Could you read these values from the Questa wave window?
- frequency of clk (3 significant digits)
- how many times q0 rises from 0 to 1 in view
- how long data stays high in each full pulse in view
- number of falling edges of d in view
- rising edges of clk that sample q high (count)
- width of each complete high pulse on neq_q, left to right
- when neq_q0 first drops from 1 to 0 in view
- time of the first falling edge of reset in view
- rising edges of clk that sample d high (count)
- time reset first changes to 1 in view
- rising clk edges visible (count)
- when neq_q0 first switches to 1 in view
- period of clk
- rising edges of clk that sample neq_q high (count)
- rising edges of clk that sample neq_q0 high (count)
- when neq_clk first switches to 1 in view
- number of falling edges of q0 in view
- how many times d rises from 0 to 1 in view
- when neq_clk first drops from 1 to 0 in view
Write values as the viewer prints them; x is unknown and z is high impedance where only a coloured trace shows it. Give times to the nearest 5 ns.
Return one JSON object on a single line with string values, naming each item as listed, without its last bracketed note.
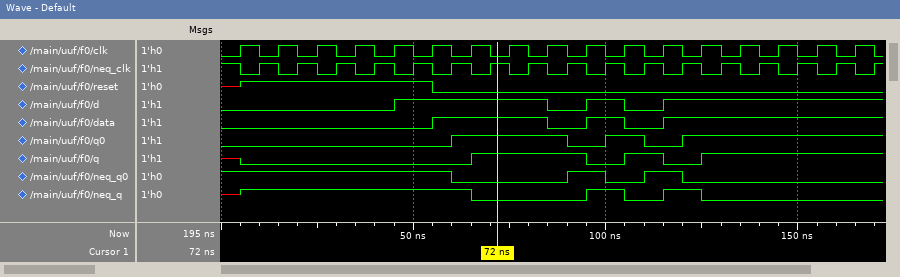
{"frequency of clk": "100 MHz", "how many times q0 rises from 0 to 1 in view": "3", "how long data stays high in each full pulse in view": "30 ns, 10 ns", "number of falling edges of d in view": "2", "rising edges of clk that sample q high": "8", "width of each complete high pulse on neq_q, left to right": "10 ns, 10 ns", "when neq_q0 first drops from 1 to 0 in view": "60 ns", "time of the first falling edge of reset in view": "55 ns", "rising edges of clk that sample d high": "10", "time reset first changes to 1 in view": "5 ns", "rising clk edges visible": "17", "when neq_q0 first switches to 1 in view": "90 ns", "period of clk": "10 ns", "rising edges of clk that sample neq_q high": "8", "rising edges of clk that sample neq_q0 high": "8", "when neq_clk first switches to 1 in view": "10 ns", "number of falling edges of q0 in view": "2", "how many times d rises from 0 to 1 in view": "3", "when neq_clk first drops from 1 to 0 in view": "5 ns"}
